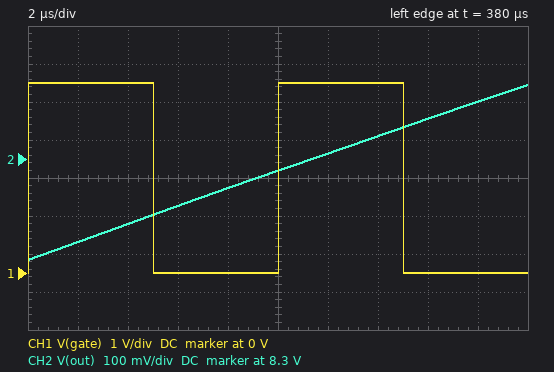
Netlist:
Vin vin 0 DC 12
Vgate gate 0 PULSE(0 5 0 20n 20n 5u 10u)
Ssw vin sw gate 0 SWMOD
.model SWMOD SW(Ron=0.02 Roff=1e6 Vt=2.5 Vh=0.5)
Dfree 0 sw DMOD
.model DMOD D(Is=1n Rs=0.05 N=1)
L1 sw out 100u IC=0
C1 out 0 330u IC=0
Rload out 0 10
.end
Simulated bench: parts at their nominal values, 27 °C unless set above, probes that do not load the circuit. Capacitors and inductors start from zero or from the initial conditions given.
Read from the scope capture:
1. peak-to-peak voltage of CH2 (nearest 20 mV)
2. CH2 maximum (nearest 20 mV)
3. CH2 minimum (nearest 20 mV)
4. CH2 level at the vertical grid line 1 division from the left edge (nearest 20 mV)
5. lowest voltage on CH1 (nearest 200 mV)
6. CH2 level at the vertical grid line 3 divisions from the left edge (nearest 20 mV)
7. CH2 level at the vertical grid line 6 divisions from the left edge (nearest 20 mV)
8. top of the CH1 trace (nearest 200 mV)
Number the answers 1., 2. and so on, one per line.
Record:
1. 460 mV
2. 8.50 V
3. 8.04 V
4. 8.08 V
5. 0 V
6. 8.18 V
7. 8.32 V
8. 5.0 V
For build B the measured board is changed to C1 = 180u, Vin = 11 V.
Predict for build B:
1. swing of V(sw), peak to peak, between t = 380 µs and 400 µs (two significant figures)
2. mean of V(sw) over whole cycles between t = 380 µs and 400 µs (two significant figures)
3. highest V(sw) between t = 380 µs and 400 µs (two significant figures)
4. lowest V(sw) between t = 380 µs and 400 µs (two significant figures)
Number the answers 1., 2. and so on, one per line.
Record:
1. 12 V
2. 5.2 V
3. 11 V
4. -690 mV
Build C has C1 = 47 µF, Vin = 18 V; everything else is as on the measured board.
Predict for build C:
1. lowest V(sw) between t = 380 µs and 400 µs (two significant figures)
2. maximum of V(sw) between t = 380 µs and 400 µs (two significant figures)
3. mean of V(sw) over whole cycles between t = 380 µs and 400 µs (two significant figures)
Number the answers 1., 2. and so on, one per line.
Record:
1. -530 mV
2. 18 V
3. 11 V
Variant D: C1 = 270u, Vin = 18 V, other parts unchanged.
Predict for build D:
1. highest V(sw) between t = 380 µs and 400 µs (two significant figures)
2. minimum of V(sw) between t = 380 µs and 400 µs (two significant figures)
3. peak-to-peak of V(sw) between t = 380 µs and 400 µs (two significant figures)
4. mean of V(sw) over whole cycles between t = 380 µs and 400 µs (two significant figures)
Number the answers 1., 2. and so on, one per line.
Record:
1. 18 V
2. -1.1 V
3. 19 V
4. 8.4 V
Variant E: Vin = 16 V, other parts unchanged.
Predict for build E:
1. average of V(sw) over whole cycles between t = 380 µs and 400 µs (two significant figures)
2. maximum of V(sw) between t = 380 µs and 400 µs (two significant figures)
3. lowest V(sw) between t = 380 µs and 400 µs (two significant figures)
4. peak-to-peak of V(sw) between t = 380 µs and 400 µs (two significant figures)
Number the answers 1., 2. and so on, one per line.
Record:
1. 7.3 V
2. 16 V
3. -1.2 V
4. 17 V
